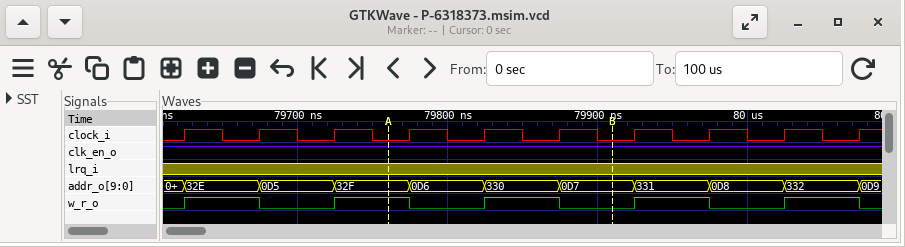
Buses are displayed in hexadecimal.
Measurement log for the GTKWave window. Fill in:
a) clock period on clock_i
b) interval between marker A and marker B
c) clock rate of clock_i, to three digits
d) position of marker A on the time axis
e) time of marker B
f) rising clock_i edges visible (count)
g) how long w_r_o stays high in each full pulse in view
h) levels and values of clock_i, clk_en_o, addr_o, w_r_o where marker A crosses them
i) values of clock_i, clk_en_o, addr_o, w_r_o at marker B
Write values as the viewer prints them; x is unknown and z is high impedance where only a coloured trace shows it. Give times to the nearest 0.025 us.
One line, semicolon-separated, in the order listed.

0.05 us; 0.15 us; 20.0 MHz; 79.75 us; 79.9 us; 10; 0.05 us, 0.05 us, 0.05 us, 0.05 us, 0.05 us; clock_i=0, clk_en_o=1, addr_o=32F, w_r_o=1; clock_i=0, clk_en_o=1, addr_o=0D7, w_r_o=0
